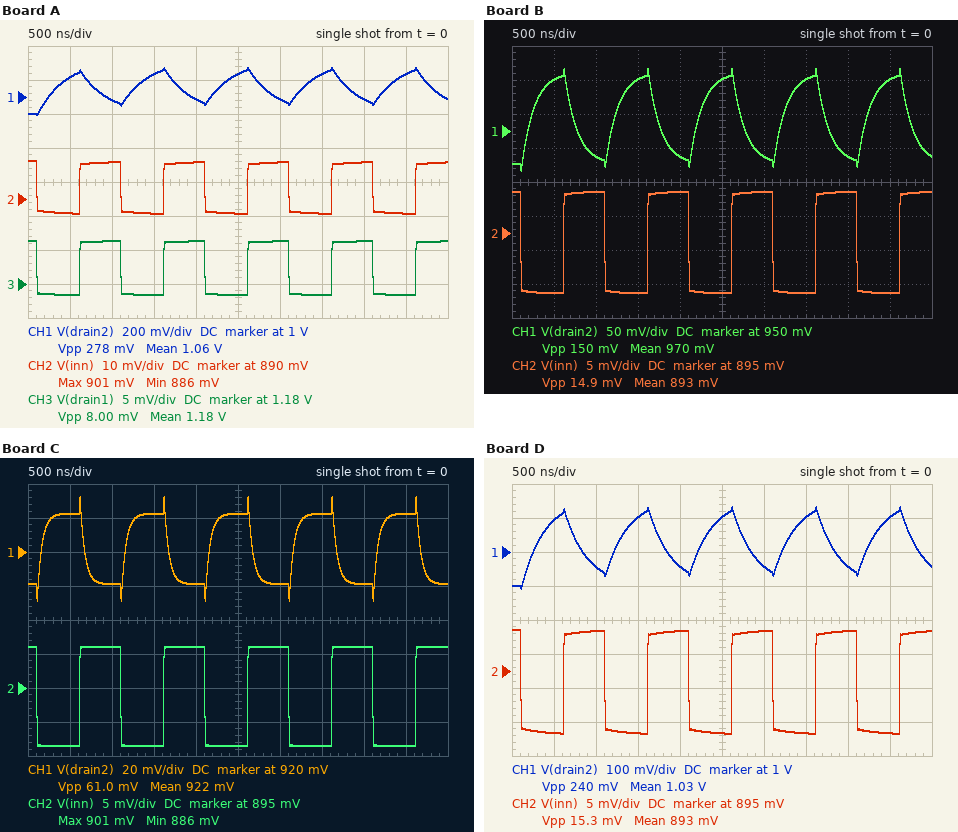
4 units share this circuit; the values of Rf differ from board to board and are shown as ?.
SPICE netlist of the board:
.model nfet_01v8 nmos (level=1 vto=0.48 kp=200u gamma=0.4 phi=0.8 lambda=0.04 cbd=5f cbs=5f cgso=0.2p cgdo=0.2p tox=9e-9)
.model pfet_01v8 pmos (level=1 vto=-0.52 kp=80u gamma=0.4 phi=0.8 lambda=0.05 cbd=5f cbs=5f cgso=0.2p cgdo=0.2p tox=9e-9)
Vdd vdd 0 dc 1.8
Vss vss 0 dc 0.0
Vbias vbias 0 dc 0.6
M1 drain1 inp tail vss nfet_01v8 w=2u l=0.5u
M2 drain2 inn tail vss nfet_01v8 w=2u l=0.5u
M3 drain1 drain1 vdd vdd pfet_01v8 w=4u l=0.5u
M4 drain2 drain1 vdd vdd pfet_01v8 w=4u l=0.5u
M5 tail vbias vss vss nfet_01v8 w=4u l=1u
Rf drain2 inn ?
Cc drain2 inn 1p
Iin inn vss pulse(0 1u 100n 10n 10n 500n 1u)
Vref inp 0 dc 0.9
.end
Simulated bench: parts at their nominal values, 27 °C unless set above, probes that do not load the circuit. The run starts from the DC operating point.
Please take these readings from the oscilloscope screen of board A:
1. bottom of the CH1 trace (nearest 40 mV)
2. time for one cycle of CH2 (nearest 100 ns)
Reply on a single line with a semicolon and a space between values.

880 mV; 1.0 µs
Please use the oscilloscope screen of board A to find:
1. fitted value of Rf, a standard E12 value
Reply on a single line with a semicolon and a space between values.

330 kΩ
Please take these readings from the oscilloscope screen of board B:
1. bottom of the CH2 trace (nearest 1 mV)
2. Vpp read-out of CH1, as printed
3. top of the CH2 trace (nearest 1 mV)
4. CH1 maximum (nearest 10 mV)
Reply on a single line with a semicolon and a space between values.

886 mV; 150 mV; 901 mV; 1.04 V
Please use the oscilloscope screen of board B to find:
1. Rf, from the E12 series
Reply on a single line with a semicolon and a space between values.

150 kΩ
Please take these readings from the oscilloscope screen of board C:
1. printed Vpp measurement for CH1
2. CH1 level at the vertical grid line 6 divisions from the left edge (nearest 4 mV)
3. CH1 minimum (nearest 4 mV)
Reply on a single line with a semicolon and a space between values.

61.0 mV; 900 mV; 892 mV
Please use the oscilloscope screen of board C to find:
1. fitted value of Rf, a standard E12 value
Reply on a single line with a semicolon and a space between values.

56 kΩ
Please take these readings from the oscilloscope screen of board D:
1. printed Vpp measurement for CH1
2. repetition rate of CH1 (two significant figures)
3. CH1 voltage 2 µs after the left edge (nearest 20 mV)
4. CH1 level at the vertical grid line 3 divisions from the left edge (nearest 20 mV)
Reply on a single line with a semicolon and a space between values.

240 mV; 1.0 MHz; 960 mV; 1.10 V
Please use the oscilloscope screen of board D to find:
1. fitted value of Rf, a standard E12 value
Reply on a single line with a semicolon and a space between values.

270 kΩ
